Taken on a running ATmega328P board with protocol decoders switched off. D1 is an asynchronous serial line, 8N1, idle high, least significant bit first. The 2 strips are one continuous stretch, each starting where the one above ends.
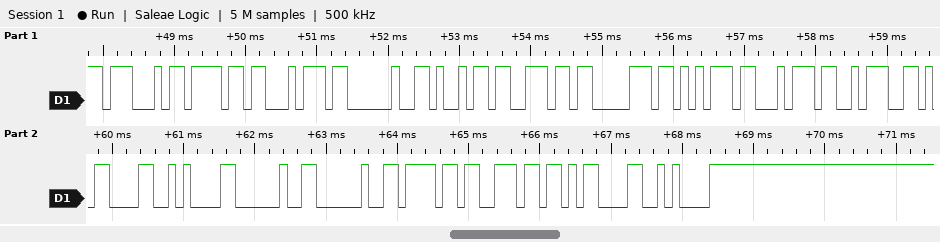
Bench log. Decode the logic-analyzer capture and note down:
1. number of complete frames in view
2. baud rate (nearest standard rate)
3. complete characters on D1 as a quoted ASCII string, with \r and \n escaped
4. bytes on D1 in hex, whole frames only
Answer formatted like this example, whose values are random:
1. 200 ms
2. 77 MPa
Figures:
1. 18
2. 9600 baud
3. "Got input:\r\n  on\r\n"
4. 47 6F 74 20 69 6E 70 75 74 3A 0D 0A 20 20 6F 6E 0D 0A
